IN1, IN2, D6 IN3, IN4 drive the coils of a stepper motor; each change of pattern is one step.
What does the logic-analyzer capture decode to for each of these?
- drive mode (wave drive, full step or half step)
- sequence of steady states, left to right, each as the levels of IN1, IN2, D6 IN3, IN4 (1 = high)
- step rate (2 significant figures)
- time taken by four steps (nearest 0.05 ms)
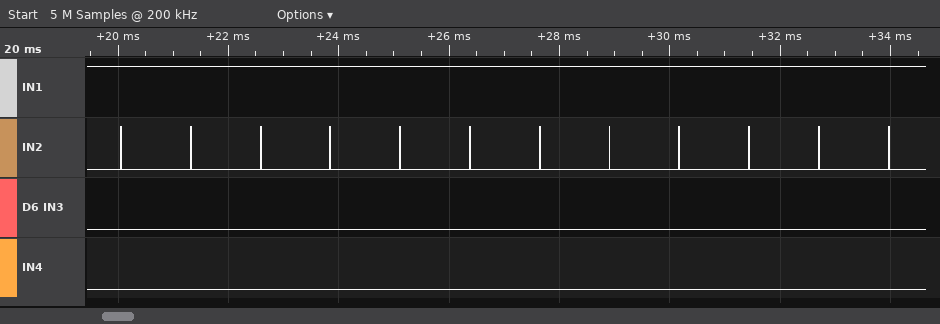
wave drive
1000 1000 1000 1000 1000 1000 1000 1000 1000 1000 1000 1000 1000
790 steps/s
5.05 ms
